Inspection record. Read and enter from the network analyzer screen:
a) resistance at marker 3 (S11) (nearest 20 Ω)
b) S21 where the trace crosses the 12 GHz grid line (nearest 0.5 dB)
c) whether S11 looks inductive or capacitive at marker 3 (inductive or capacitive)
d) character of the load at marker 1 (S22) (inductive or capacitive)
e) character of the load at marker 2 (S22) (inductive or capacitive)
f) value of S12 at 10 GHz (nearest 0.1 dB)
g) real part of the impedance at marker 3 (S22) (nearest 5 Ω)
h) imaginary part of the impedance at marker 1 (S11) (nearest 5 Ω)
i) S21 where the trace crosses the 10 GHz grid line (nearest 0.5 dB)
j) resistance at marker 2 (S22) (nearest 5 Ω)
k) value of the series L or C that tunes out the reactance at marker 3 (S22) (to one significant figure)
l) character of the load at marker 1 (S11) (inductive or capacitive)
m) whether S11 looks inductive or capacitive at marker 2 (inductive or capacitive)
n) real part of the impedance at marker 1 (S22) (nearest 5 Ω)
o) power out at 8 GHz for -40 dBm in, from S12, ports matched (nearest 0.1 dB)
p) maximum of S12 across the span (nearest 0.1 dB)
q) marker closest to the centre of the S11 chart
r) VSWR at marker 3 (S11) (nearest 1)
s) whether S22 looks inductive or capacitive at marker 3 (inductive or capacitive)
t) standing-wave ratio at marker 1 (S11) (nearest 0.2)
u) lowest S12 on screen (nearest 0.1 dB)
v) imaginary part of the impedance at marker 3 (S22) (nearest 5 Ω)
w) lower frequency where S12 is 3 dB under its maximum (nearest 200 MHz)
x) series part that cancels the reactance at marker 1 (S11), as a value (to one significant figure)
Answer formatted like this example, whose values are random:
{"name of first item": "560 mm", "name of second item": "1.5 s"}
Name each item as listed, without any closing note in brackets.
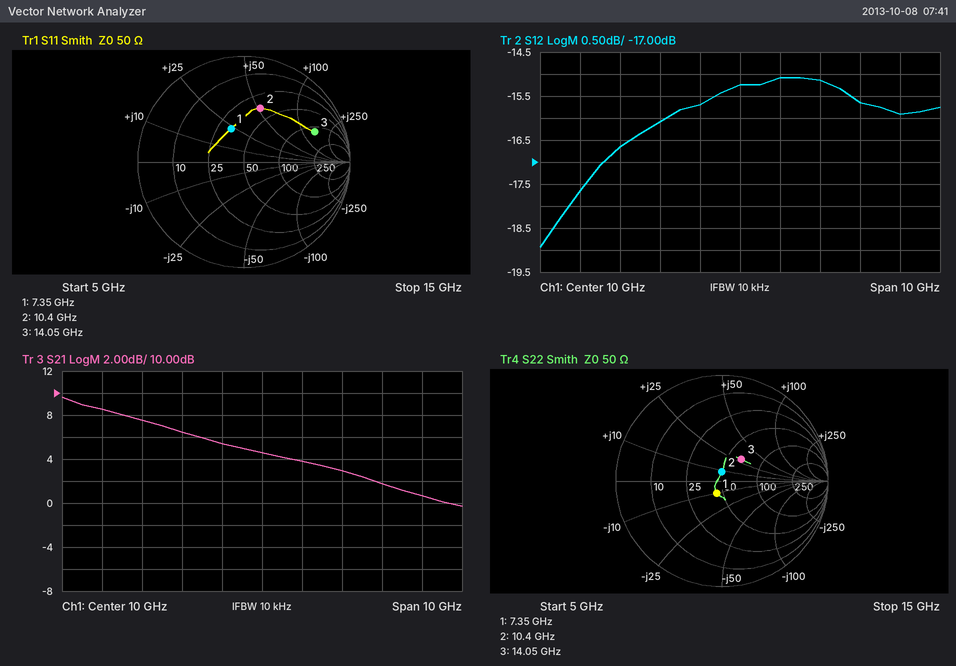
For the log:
{"resistance at marker 3 (S11)": "120 Ω", "S21 where the trace crosses the 12 GHz grid line": "3.0 dB", "whether S11 looks inductive or capacitive at marker 3": "inductive", "character of the load at marker 1 (S22)": "capacitive", "character of the load at marker 2 (S22)": "inductive", "value of S12 at 10 GHz": "-15.2 dB", "real part of the impedance at marker 3 (S22)": "65 Ω", "imaginary part of the impedance at marker 1 (S11)": "+25 Ω", "S21 where the trace crosses the 10 GHz grid line": "4.5 dB", "resistance at marker 2 (S22)": "50 Ω", "value of the series L or C that tunes out the reactance at marker 3 (S22)": "400 fF", "character of the load at marker 1 (S11)": "inductive", "whether S11 looks inductive or capacitive at marker 2": "inductive", "real part of the impedance at marker 1 (S22)": "45 Ω", "power out at 8 GHz for -40 dBm in, from S12, ports matched": "-56.1 dBm", "maximum of S12 across the span": "-15.1 dB", "marker closest to the centre of the S11 chart": "marker 1", "VSWR at marker 3 (S11)": "6", "whether S22 looks inductive or capacitive at marker 3": "inductive", "standing-wave ratio at marker 1 (S11)": "2.0", "lowest S12 on screen": "-18.9 dB", "imaginary part of the impedance at marker 3 (S22)": "+30 Ω", "lower frequency where S12 is 3 dB under its maximum": "5.6 GHz", "series part that cancels the reactance at marker 1 (S11), as a value": "900 fF"}
